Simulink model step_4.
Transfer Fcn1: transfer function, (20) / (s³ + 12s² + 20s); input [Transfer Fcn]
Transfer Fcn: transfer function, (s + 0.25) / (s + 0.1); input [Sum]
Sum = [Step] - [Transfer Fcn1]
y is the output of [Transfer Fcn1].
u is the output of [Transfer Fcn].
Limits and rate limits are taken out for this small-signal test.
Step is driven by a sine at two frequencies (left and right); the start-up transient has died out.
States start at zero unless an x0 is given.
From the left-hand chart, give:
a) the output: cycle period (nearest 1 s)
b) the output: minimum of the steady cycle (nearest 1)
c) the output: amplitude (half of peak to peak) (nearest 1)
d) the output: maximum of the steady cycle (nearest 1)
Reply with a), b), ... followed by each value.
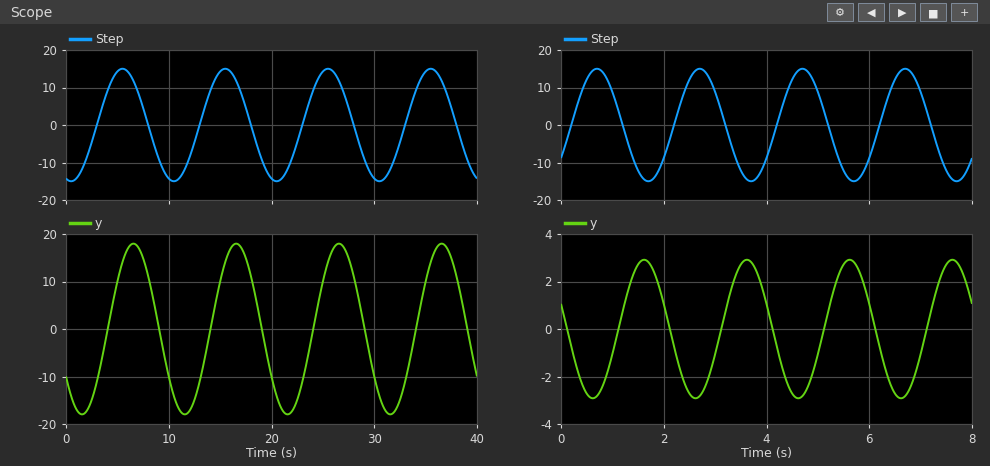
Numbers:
a) 10 s
b) -18
c) 18
d) 18
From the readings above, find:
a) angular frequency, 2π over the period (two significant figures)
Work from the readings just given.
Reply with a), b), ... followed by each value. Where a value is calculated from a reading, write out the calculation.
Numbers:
a) 2π / 10 = 0.63 rad/s
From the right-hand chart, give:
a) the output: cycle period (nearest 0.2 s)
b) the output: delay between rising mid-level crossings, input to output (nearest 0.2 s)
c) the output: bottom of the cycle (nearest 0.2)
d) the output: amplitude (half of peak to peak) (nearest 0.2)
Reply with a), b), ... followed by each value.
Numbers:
a) 2.0 s
b) 1.0 s
c) -3.0
d) 3.0
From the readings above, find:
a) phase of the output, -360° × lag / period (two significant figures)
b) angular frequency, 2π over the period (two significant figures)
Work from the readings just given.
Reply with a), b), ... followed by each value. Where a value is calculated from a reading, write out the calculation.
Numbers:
a) -360 × 1 / 2 = -180°
b) 2π / 2 = 3.1 rad/s
